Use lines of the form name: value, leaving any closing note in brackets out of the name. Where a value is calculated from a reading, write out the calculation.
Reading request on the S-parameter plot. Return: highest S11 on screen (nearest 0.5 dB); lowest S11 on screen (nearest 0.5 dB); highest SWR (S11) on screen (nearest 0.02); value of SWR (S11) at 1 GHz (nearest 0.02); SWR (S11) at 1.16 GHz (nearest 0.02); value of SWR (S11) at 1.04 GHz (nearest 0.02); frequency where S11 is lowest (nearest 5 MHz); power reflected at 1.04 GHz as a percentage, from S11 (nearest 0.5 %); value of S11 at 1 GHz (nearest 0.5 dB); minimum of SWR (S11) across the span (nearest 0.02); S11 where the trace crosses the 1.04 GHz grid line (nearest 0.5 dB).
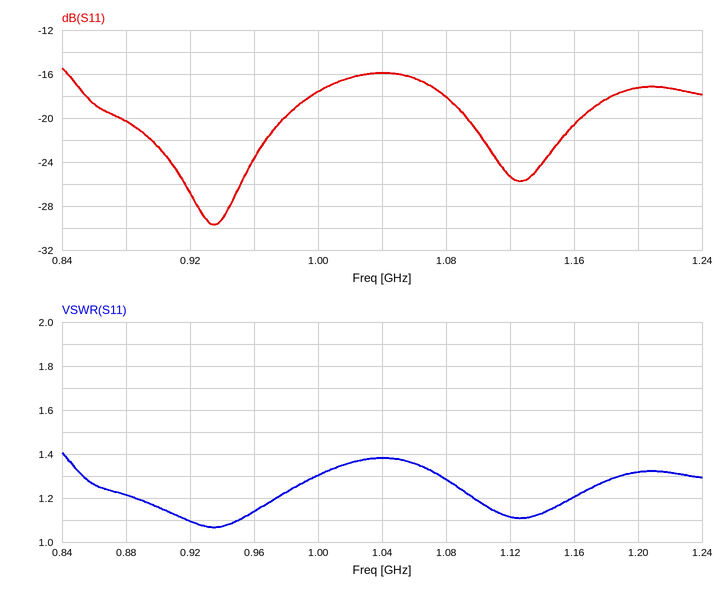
highest S11 on screen: -15.5 dB
lowest S11 on screen: -29.5 dB
highest SWR (S11) on screen: 1.40
value of SWR (S11) at 1 GHz: 1.30
SWR (S11) at 1.16 GHz: 1.20
value of SWR (S11) at 1.04 GHz: 1.38
frequency where S11 is lowest: 935 MHz
power reflected at 1.04 GHz as a percentage, from S11: 10^(-16/10) ≈ 2.5 %
value of S11 at 1 GHz: -17.5 dB
minimum of SWR (S11) across the span: 1.06
S11 where the trace crosses the 1.04 GHz grid line: -16.0 dB
